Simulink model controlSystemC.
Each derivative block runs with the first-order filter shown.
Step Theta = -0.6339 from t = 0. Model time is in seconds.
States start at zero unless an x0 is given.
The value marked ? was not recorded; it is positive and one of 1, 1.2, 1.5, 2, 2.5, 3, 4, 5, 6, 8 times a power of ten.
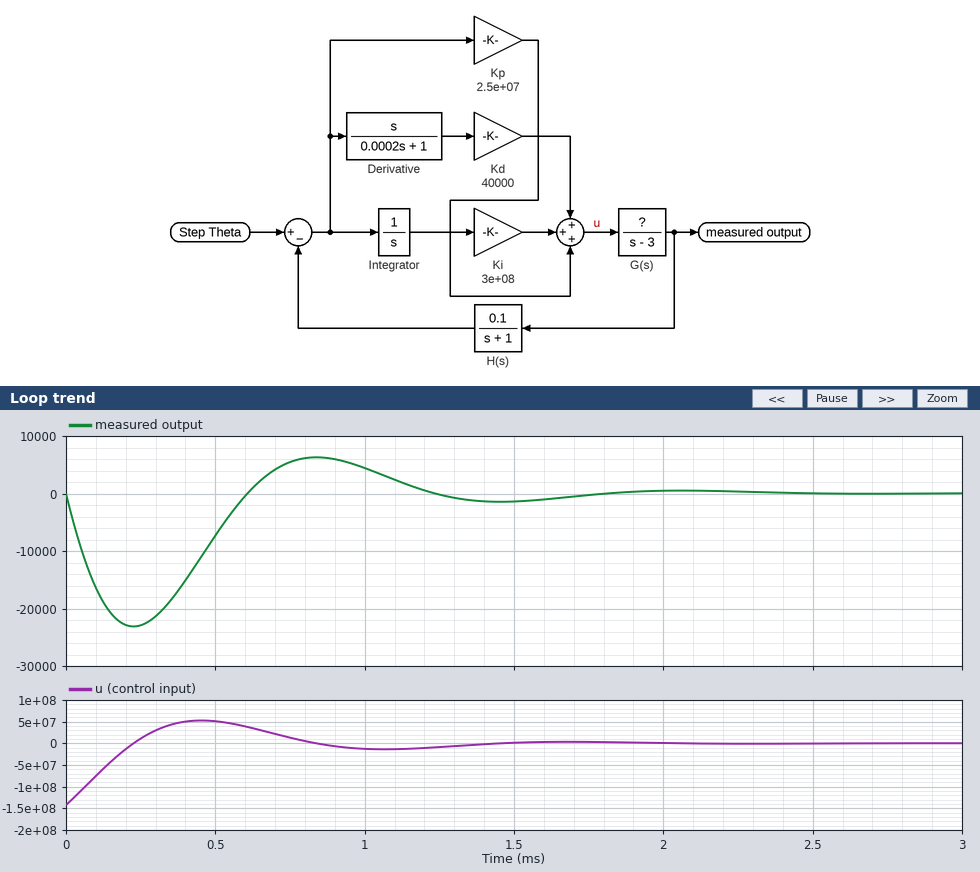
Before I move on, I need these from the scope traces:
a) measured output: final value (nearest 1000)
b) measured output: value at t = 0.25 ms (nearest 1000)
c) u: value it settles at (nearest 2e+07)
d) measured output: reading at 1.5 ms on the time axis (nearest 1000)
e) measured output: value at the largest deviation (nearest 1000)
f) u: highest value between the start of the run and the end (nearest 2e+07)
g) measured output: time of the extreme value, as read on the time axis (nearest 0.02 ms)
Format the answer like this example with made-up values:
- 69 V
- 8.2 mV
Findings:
- 0
- -23000
- 0
- -1000
- -23000
- 60000000
- 0.22 ms
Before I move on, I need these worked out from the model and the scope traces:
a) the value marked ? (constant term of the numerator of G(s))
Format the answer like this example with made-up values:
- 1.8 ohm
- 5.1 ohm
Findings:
- 1.5
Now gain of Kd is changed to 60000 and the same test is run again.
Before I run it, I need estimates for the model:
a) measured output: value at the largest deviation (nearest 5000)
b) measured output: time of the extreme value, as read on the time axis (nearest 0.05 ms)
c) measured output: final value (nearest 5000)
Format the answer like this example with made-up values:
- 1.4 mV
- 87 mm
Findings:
- -30000
- 0.20 ms
- 0
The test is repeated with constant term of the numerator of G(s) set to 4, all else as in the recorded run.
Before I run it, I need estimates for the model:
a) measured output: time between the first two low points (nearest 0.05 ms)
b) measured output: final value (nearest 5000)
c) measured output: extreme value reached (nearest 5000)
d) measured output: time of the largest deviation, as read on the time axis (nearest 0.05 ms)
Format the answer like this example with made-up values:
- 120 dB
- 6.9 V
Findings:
- 0.70 ms
- 0
- -45000
- 0.15 ms
